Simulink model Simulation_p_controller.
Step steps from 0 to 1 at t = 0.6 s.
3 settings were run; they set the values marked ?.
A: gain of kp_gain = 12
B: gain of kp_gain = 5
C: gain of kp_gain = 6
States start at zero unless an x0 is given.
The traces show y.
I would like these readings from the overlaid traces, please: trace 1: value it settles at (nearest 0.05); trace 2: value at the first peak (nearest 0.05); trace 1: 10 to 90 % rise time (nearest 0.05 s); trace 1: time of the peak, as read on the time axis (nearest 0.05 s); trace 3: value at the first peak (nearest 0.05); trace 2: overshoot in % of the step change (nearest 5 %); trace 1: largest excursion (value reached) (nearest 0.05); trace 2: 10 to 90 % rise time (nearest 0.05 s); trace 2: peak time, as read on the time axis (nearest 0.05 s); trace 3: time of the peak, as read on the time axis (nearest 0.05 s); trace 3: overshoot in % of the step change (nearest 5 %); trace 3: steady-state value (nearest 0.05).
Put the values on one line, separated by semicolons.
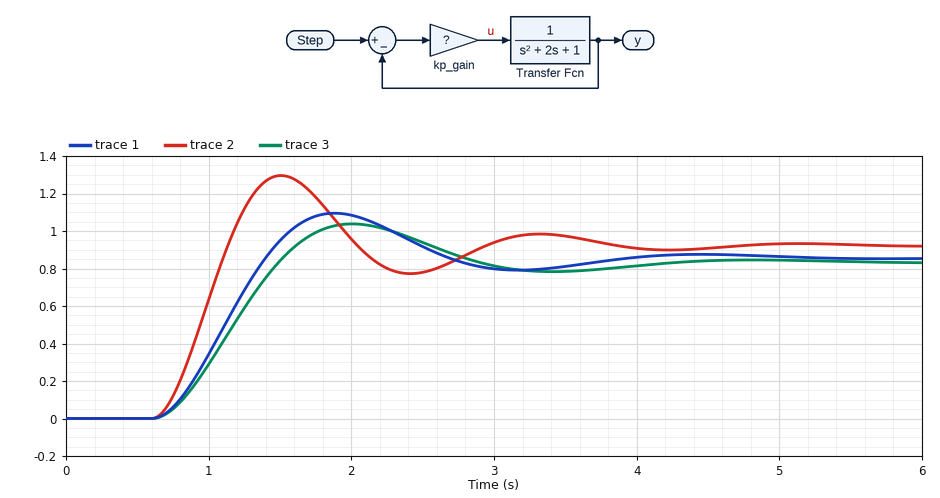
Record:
0.85; 1.30; 0.55 s; 1.90 s; 1.05; 40 %; 1.10; 0.35 s; 1.50 s; 2.00 s; 25 %; 0.85
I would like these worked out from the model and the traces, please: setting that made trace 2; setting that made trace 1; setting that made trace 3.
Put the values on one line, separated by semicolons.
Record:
A; C; B
